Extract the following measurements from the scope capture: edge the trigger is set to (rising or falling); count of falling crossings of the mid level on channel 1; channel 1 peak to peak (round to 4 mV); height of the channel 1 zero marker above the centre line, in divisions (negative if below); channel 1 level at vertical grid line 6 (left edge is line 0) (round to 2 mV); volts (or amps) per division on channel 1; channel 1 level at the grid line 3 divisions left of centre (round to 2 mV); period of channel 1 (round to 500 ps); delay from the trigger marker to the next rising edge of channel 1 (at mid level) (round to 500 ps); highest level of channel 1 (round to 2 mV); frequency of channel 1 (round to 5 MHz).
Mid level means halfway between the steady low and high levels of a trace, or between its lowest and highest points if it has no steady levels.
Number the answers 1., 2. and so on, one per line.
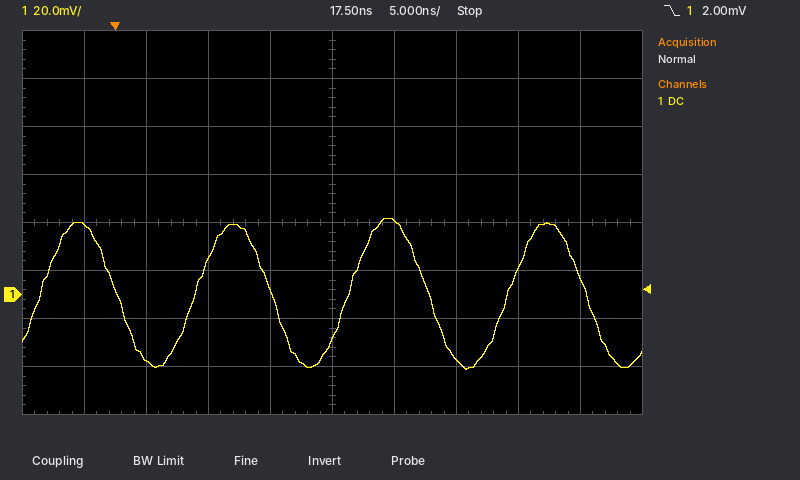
1. falling
2. 4
3. 64 mV
4. -1.5 div
5. 30 mV
6. 20 mV
7. -28 mV
8. 12.5 ns
9. 6.5 ns
10. 32 mV
11. 80 MHz
